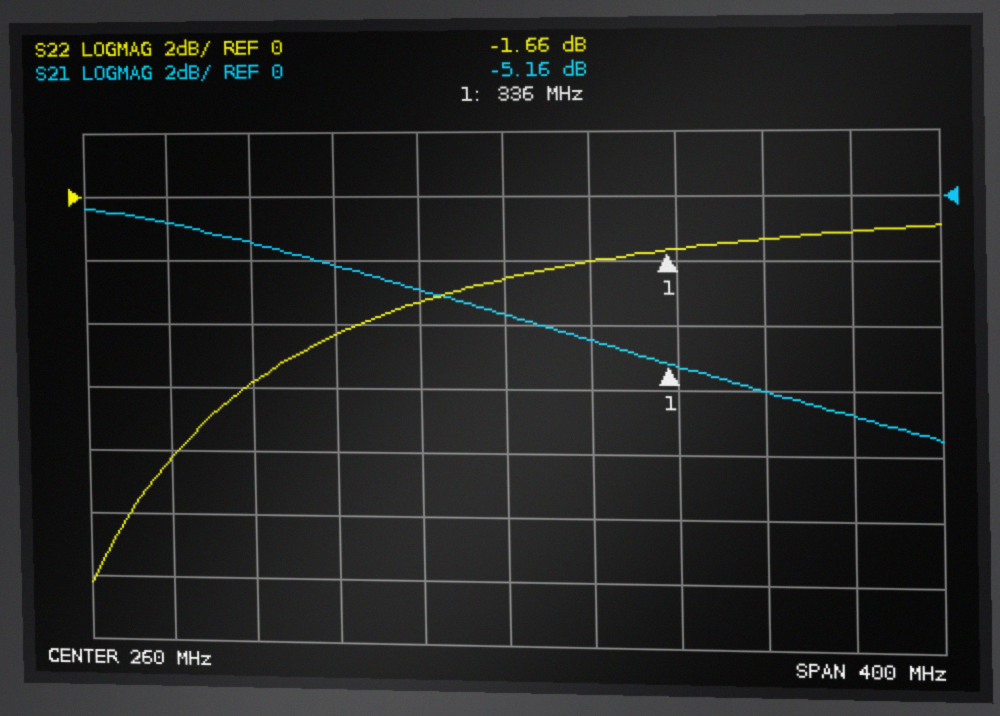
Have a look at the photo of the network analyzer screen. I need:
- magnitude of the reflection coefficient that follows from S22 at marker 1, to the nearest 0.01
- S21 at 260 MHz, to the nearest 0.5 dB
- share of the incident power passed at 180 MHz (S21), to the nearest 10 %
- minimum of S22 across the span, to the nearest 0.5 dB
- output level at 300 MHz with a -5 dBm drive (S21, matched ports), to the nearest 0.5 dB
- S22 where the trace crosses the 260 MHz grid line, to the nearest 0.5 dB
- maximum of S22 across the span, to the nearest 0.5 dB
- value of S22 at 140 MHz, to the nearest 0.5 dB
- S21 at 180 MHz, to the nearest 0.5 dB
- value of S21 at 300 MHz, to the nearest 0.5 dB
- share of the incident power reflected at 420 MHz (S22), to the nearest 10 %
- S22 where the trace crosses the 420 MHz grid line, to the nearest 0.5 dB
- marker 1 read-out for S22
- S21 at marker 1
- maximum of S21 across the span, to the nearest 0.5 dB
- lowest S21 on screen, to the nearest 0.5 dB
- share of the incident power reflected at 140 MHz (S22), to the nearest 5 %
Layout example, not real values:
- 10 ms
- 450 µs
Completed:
- 0.83
- -3.5 dB
- 60 %
- -12.0 dB
- -9.5 dBm
- -2.5 dB
- -1.0 dB
- -6.0 dB
- -2.0 dB
- -4.5 dB
- 80 %
- -1.0 dB
- -1.66 dB
- -5.16 dB
- -0.5 dB
- -7.5 dB
- 25 %
